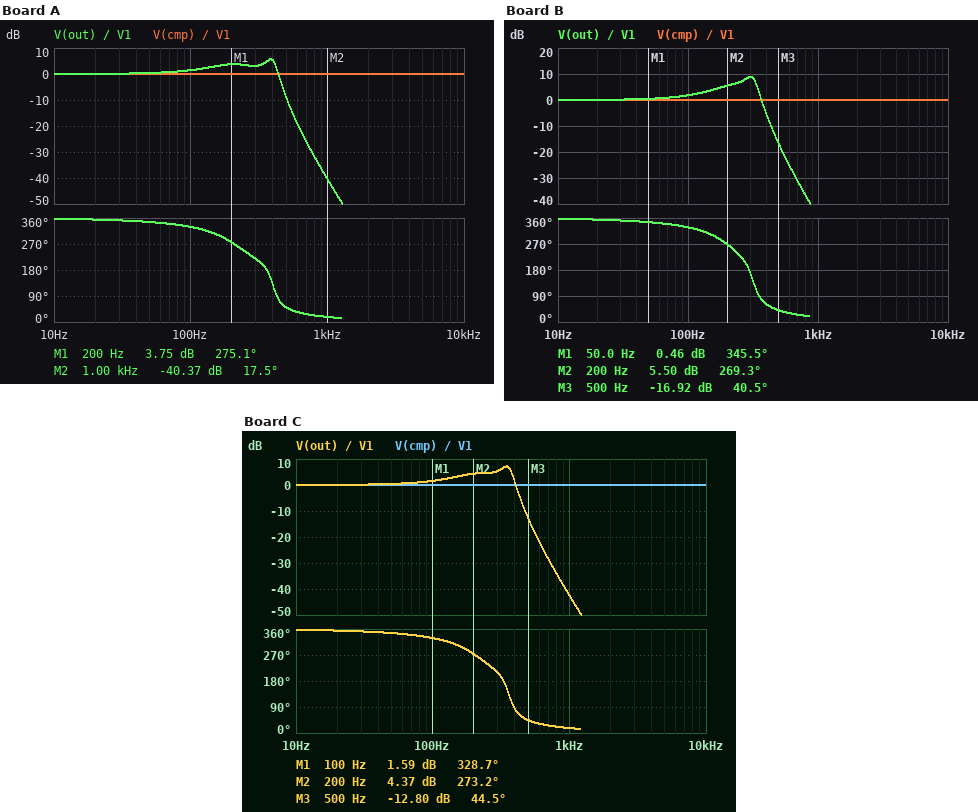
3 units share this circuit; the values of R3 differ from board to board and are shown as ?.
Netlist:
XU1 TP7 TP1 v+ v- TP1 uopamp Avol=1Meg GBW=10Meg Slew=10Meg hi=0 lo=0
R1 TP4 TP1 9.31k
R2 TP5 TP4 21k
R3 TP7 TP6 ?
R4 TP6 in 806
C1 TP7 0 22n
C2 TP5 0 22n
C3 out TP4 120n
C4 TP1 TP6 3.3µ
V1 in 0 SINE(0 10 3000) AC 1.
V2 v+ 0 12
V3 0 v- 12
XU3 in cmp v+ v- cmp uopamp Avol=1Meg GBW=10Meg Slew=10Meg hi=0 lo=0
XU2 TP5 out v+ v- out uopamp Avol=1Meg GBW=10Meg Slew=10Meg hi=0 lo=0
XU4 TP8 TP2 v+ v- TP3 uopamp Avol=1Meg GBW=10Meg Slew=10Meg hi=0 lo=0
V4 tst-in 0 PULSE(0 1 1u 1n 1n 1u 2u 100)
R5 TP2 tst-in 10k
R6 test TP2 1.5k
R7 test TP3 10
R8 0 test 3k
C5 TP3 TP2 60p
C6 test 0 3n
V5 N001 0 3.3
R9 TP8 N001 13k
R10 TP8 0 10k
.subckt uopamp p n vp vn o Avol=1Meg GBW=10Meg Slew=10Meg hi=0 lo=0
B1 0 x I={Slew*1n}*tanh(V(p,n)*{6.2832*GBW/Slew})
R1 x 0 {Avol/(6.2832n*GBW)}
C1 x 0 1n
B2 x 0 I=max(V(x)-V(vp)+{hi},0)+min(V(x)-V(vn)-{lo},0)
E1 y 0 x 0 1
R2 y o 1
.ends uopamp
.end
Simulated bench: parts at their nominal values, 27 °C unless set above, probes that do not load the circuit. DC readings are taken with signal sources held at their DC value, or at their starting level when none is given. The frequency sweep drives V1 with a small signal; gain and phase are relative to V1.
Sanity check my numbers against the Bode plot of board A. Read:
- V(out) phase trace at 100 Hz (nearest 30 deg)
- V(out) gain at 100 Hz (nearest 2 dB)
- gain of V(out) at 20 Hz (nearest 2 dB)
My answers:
330 deg
2 dB
0 dB
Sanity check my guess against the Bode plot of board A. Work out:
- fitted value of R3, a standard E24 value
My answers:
2.7 kΩ
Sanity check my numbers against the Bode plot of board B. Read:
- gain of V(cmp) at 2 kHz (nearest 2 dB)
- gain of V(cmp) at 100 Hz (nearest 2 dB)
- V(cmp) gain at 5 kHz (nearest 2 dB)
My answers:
0 dB
0 dB
0 dB
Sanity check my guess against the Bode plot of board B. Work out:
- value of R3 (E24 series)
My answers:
4.3 kΩ
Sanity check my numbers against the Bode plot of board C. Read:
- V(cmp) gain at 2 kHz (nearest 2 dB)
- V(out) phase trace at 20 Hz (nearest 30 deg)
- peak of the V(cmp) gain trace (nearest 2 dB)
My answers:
0 dB
360 deg
0 dB
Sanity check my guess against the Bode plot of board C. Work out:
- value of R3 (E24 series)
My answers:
3.3 kΩ
